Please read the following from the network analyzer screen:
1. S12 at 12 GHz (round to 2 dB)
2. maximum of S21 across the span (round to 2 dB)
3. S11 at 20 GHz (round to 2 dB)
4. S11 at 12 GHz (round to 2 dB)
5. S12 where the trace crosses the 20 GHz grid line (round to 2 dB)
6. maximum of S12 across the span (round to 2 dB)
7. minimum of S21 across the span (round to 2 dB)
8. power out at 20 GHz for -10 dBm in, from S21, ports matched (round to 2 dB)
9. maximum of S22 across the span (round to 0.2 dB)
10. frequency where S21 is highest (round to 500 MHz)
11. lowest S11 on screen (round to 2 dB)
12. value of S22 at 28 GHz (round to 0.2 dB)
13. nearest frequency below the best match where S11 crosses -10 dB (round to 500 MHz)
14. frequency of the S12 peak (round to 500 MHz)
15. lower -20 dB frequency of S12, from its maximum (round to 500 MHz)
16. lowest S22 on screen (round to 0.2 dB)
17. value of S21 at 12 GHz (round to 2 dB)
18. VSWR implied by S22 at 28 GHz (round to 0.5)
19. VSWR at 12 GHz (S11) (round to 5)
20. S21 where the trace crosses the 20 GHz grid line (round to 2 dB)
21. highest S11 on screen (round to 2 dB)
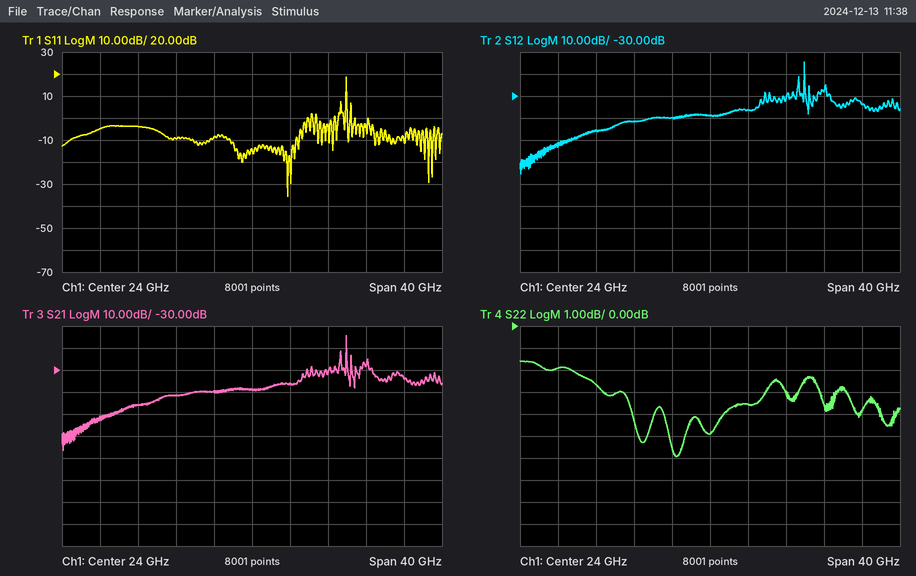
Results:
-46 dB
-14 dB
-8 dB
-4 dB
-40 dB
-14 dB
-66 dB
-50 dBm
-1.6 dB
34.0 GHz
-36 dB
-3.6 dB
21.5 GHz
34.0 GHz
29.0 GHz
-6.0 dB
-46 dB
5.0
5
-40 dB
18 dB
